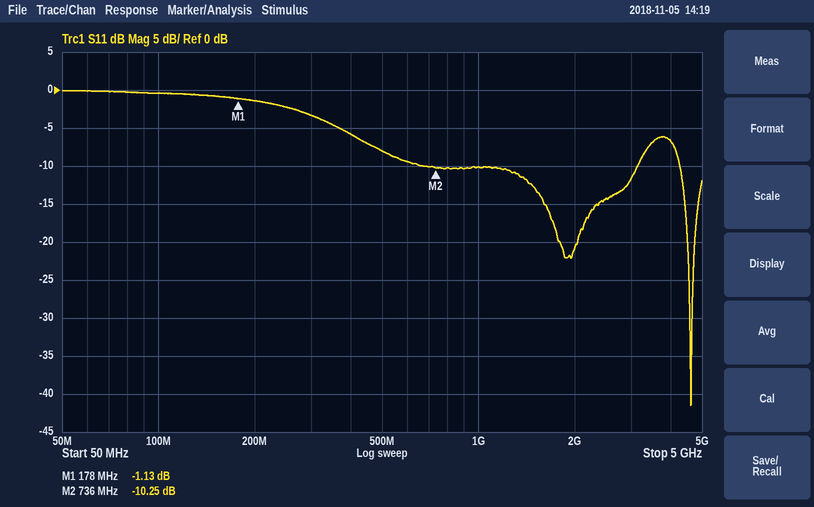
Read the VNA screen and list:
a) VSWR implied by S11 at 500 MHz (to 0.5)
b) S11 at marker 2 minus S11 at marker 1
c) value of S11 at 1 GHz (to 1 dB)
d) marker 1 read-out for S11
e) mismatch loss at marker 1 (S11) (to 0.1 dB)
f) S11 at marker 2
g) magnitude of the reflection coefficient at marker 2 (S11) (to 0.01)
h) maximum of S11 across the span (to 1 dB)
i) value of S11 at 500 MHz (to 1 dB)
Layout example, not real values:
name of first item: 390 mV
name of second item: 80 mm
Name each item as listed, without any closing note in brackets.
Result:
VSWR implied by S11 at 500 MHz: 2.5
S11 at marker 2 minus S11 at marker 1: -9.12 dB
value of S11 at 1 GHz: -10 dB
marker 1 read-out for S11: -1.13 dB
mismatch loss at marker 1 (S11): 6.4 dB
S11 at marker 2: -10.25 dB
magnitude of the reflection coefficient at marker 2 (S11): 0.31
maximum of S11 across the span: 0 dB
value of S11 at 500 MHz: -8 dB
